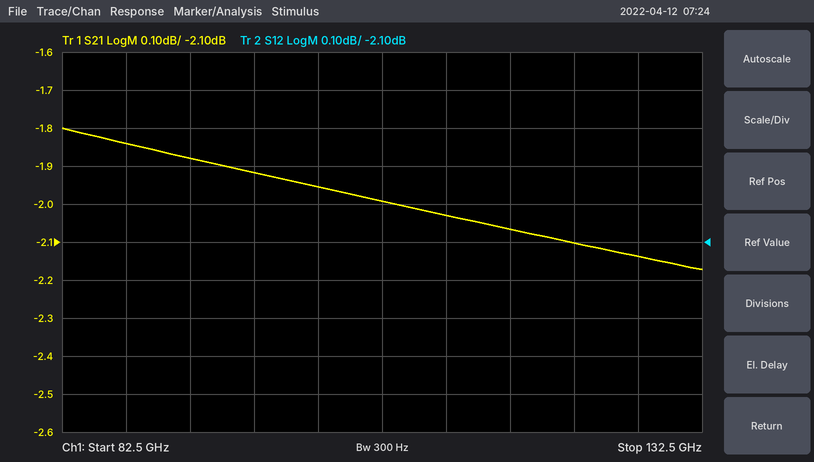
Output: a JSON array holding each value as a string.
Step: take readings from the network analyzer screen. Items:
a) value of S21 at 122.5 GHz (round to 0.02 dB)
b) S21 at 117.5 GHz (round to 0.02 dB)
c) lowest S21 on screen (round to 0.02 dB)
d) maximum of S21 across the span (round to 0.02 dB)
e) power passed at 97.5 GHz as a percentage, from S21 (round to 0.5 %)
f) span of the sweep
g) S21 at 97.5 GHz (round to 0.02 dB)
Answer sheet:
["-2.10 dB", "-2.06 dB", "-2.18 dB", "-1.80 dB", "64.5 %", "50 GHz", "-1.92 dB"]
